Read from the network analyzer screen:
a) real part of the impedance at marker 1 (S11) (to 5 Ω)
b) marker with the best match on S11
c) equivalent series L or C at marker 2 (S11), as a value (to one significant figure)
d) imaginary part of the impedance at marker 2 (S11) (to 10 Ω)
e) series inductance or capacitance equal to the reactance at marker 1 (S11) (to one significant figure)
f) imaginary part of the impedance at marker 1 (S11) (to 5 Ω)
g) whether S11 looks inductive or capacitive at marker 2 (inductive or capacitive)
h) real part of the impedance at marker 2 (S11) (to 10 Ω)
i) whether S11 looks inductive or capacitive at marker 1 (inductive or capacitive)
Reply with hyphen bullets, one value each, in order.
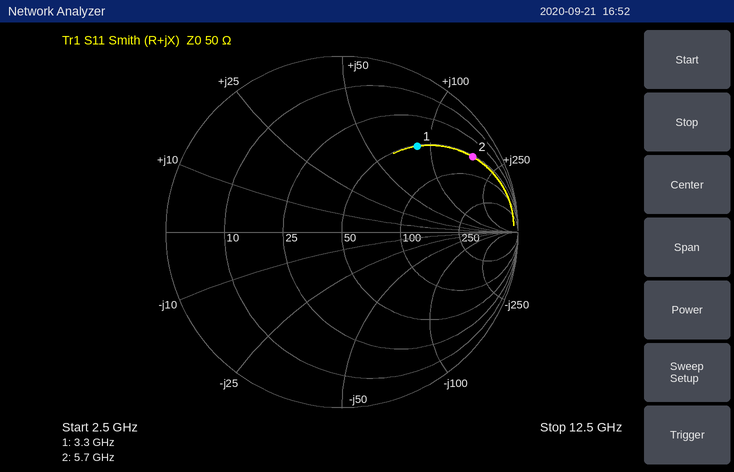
- 50 Ω
- marker 1
- 5 nH
- +170 Ω
- 4 nH
- +85 Ω
- inductive
- 50 Ω
- inductive
